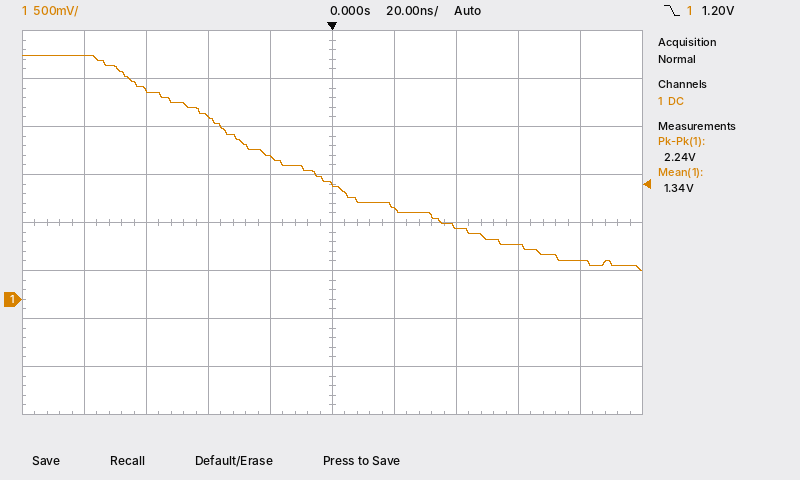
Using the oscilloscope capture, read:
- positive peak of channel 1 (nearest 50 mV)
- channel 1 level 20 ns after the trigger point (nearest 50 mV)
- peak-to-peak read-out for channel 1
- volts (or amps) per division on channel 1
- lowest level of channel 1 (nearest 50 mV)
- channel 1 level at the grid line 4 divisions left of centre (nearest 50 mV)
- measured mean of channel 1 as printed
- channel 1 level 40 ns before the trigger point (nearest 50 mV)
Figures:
2.55 V
950 mV
2.24 V
500 mV
300 mV
2.55 V
1.34 V
1.90 V
